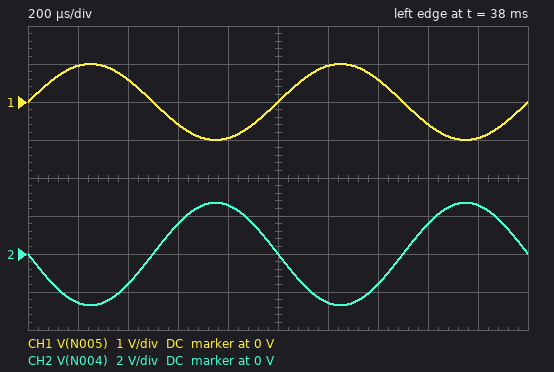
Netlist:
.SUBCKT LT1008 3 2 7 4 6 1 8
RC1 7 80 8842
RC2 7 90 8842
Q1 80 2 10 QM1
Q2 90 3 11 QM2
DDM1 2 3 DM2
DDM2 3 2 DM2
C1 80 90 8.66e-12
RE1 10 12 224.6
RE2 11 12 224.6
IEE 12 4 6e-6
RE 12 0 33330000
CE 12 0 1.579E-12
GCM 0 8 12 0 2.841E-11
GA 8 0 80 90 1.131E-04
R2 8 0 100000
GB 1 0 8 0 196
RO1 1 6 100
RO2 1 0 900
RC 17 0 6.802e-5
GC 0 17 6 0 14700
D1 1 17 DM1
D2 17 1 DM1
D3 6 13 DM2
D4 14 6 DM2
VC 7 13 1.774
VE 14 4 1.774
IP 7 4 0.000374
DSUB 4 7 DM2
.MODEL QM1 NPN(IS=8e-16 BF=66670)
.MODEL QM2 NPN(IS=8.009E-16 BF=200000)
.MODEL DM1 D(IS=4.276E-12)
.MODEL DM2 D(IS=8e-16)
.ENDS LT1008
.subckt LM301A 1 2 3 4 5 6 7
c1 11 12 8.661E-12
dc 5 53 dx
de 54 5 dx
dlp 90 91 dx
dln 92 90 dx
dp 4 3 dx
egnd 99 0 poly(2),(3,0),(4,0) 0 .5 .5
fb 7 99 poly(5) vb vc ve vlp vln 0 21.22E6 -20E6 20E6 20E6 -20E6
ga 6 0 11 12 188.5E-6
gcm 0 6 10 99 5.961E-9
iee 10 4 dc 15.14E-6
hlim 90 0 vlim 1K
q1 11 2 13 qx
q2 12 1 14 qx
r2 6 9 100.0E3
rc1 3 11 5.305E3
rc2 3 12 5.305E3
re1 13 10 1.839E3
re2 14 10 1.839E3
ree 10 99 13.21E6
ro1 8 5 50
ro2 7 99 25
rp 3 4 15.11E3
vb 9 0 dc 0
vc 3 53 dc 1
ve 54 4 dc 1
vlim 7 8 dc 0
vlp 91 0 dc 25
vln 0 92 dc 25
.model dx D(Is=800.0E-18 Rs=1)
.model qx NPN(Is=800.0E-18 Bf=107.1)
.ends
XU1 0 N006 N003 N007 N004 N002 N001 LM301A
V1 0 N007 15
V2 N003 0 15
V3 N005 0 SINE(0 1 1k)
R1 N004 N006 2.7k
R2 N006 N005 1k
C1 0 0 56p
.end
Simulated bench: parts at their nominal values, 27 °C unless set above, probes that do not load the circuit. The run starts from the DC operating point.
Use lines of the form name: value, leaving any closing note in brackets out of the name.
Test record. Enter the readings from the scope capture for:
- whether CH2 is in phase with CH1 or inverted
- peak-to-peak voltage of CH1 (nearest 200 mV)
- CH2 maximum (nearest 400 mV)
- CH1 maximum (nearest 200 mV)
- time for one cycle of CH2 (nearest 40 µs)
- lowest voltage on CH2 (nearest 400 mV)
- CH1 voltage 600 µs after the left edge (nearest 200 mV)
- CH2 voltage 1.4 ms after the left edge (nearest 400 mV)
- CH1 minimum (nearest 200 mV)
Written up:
whether CH2 is in phase with CH1 or inverted: inverted
peak-to-peak voltage of CH1: 2.0 V
CH2 maximum: 2.8 V
CH1 maximum: 1.0 V
time for one cycle of CH2: 1.00 ms
lowest voltage on CH2: -2.8 V
CH1 voltage 600 µs after the left edge: -600 mV
CH2 voltage 1.4 ms after the left edge: -1.6 V
CH1 minimum: -1.0 V
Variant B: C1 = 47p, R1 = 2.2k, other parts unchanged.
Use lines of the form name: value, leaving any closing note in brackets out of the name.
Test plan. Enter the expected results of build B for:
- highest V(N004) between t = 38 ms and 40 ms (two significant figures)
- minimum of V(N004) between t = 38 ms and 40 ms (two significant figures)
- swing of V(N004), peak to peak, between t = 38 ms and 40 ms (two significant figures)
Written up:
highest V(N004) between t = 38 ms and 40 ms: 2.2 V
minimum of V(N004) between t = 38 ms and 40 ms: -2.2 V
swing of V(N004), peak to peak, between t = 38 ms and 40 ms: 4.4 V
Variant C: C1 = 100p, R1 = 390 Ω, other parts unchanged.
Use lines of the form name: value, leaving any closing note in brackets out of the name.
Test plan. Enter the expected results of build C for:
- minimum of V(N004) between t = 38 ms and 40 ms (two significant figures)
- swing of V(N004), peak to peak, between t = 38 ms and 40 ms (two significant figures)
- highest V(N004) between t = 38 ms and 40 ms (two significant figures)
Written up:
minimum of V(N004) between t = 38 ms and 40 ms: -390 mV
swing of V(N004), peak to peak, between t = 38 ms and 40 ms: 780 mV
highest V(N004) between t = 38 ms and 40 ms: 390 mV
